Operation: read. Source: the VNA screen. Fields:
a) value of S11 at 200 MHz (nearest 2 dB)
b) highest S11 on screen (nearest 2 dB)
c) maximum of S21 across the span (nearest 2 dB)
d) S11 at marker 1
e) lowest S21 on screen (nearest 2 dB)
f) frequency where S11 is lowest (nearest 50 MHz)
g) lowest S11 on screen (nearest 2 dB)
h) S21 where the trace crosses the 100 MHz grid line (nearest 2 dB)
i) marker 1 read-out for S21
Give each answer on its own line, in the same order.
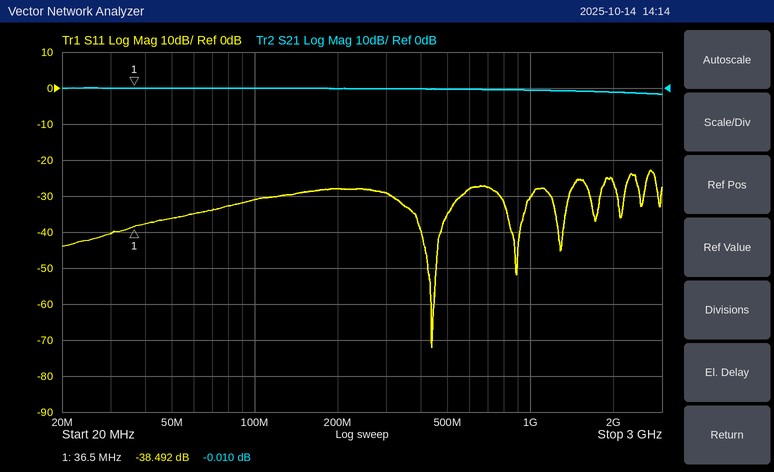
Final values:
-28 dB
-22 dB
0 dB
-38.492 dB
-2 dB
450 MHz
-72 dB
0 dB
-0.010 dB
